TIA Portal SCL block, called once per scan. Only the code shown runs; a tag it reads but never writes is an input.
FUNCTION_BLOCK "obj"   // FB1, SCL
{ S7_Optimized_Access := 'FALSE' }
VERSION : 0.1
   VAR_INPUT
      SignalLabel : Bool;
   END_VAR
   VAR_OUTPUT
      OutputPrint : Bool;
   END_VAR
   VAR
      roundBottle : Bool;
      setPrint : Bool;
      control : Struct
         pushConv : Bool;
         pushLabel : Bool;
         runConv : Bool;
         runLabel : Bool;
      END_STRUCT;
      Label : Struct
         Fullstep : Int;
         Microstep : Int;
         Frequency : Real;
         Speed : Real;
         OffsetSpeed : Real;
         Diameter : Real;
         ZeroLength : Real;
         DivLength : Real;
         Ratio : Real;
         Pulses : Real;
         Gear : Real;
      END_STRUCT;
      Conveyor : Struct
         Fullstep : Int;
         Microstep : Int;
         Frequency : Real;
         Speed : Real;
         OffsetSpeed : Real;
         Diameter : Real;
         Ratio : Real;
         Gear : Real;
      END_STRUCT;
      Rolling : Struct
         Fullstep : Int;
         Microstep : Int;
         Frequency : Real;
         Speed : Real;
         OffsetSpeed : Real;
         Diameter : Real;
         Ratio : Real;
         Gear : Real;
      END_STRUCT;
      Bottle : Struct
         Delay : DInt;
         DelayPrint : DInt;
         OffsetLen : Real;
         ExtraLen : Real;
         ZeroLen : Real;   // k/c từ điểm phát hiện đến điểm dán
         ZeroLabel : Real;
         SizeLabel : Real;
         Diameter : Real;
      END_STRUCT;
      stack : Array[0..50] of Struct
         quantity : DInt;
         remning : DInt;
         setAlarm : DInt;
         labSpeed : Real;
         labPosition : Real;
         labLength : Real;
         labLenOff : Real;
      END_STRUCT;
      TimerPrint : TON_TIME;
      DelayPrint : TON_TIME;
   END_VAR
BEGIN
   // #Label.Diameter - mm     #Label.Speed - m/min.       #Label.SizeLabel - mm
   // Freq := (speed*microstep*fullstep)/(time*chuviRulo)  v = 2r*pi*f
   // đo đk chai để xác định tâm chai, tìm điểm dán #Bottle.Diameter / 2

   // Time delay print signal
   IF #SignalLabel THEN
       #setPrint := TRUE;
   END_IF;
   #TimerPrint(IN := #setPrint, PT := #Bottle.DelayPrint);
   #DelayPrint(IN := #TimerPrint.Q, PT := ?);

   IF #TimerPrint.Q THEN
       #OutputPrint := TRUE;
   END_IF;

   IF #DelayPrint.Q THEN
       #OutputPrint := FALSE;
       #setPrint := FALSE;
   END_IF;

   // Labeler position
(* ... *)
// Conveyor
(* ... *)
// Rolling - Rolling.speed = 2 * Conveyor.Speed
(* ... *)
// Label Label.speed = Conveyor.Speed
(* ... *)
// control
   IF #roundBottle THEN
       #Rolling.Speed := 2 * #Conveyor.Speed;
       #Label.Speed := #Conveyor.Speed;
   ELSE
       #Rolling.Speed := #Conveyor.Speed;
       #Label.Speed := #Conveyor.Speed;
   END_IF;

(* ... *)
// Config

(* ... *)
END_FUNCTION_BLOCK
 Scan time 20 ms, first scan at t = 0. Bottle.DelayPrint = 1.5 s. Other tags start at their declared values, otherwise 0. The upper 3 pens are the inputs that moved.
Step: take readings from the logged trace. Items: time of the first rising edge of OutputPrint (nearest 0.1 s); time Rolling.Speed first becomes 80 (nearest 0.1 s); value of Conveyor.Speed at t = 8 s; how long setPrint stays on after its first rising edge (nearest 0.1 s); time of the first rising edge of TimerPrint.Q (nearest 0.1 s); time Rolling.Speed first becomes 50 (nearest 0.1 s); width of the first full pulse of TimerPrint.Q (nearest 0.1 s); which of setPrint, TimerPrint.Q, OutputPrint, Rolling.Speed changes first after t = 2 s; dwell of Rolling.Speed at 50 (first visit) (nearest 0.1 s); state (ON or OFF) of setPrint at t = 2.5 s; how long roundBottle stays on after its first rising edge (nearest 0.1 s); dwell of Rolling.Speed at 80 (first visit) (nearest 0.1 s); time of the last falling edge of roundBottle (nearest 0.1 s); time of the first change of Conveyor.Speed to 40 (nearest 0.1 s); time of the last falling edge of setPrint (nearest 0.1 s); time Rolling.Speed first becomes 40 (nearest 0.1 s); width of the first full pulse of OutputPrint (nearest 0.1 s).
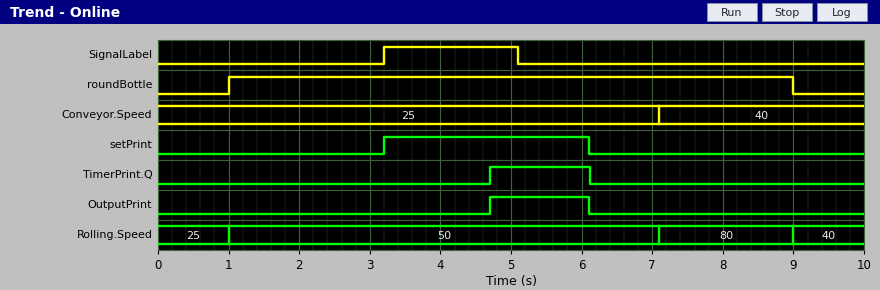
4.7 s
7.1 s
40
2.9 s
4.7 s
1.0 s
1.4 s
setPrint
6.1 s
OFF
8.0 s
1.9 s
9.0 s
7.1 s
6.1 s
9.0 s
1.4 s
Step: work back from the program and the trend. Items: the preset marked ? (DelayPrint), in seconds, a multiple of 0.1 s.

1.4 s
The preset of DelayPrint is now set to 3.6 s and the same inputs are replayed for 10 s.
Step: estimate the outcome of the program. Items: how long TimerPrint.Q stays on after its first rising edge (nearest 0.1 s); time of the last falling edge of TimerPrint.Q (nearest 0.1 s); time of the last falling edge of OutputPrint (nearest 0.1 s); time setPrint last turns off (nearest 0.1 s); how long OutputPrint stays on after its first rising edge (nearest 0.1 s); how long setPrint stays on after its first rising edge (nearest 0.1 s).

3.6 s
8.3 s
8.3 s
8.3 s
3.6 s
5.1 s
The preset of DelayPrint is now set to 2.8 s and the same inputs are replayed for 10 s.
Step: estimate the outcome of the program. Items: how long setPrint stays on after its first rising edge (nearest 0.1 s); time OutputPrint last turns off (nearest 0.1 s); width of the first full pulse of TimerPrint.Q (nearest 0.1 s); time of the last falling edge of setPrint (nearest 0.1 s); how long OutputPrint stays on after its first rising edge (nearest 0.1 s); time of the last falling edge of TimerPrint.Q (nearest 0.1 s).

4.3 s
7.5 s
2.8 s
7.5 s
2.8 s
7.5 s
